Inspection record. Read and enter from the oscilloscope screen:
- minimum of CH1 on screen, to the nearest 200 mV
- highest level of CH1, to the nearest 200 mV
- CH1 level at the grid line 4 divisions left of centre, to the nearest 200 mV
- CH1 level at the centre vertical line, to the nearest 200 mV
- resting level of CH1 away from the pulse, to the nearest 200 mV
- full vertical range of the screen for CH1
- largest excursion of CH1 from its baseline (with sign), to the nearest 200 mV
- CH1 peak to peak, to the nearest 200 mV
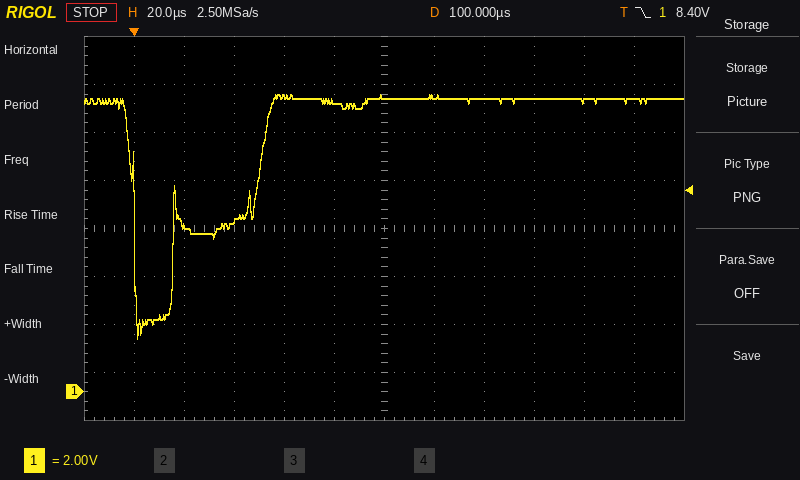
2.2 V
12.4 V
7.0 V
12.2 V
12.2 V
16 V
-10.0 V
10.2 V
